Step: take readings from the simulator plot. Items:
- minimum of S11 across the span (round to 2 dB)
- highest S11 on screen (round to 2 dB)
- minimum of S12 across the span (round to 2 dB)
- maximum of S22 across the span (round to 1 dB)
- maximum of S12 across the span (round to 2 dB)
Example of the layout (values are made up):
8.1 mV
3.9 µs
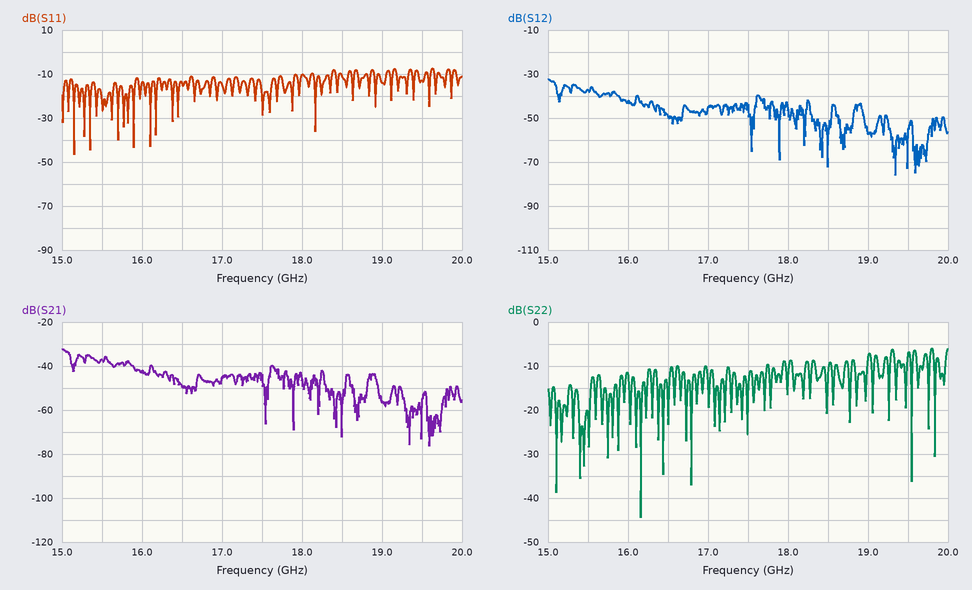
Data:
-46 dB
-8 dB
-76 dB
-6 dB
-32 dB
